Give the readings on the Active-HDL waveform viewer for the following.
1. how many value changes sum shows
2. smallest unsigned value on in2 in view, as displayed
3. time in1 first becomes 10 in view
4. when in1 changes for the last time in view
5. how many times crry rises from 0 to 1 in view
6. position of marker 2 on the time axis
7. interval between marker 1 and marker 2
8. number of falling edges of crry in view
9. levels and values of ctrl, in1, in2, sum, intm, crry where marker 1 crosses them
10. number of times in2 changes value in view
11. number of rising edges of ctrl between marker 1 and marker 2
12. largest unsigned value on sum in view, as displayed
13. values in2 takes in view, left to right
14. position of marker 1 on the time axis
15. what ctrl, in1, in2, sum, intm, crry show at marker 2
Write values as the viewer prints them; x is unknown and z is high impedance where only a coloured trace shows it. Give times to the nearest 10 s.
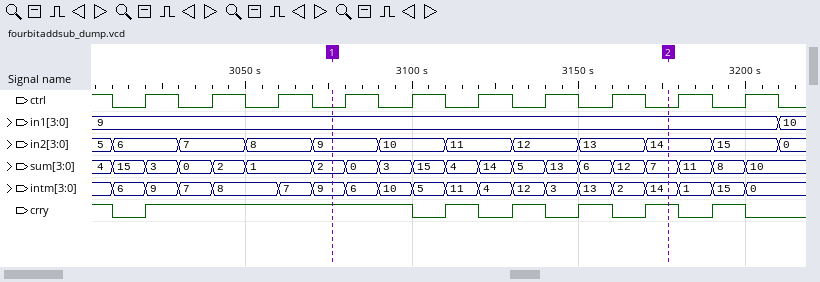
19
0
3210 s
3210 s
6
3180 s
100 s
7
ctrl=0, in1=9, in2=9, sum=2, intm=9, crry=1
11
5
15
5, 6, 7, 8, 9, 10, 11, 12, 13, 14, 15, 0
3080 s
ctrl=0, in1=9, in2=14, sum=7, intm=14, crry=1
